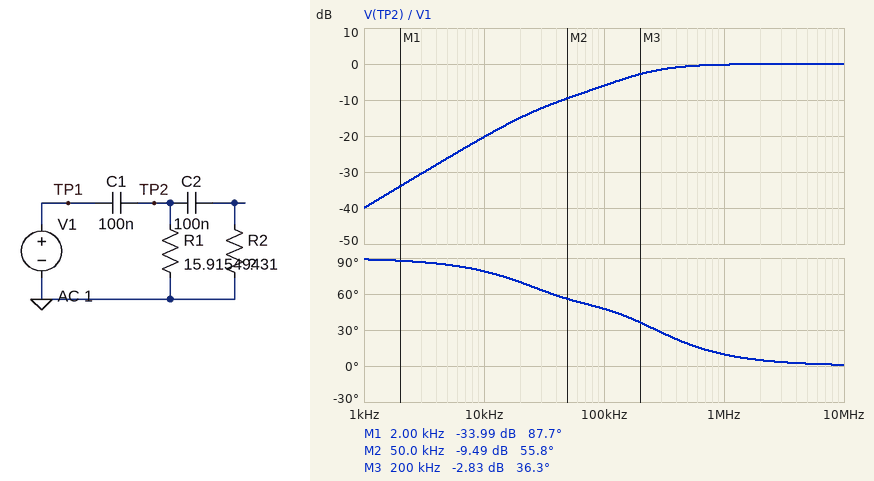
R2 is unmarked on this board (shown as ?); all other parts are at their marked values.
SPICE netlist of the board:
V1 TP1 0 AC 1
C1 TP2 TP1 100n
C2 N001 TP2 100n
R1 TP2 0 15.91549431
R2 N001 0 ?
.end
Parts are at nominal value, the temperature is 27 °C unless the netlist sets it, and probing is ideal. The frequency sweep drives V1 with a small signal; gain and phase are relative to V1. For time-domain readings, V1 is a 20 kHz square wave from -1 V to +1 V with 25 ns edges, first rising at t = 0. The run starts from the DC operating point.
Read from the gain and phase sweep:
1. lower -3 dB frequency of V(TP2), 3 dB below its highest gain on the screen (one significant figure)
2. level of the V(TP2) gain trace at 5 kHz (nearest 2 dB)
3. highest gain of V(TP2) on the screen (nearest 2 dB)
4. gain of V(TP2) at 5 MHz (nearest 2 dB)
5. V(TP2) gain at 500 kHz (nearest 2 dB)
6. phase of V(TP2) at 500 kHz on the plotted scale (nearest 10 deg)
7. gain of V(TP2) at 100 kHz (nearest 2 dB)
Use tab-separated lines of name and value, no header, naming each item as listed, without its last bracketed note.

lower -3 dB frequency of V(TP2), 3 dB below its highest gain on the screen	200 kHz
level of the V(TP2) gain trace at 5 kHz	-26 dB
highest gain of V(TP2) on the screen	0 dB
gain of V(TP2) at 5 MHz	0 dB
V(TP2) gain at 500 kHz	0 dB
phase of V(TP2) at 500 kHz on the plotted scale	20 deg
gain of V(TP2) at 100 kHz	-6 dB
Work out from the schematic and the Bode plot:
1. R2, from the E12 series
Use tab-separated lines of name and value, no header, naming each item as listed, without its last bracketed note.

R2, from the E12 series	22 Ω
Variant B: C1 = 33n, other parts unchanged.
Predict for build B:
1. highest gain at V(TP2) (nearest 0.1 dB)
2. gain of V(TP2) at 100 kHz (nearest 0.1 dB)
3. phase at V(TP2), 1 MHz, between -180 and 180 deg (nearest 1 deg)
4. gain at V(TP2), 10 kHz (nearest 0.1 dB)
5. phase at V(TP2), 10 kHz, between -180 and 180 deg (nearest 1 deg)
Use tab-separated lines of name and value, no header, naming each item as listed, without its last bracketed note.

highest gain at V(TP2)	0 dB
gain of V(TP2) at 100 kHz	-13.8 dB
phase at V(TP2), 1 MHz, between -180 and 180 deg	27 deg
gain at V(TP2), 10 kHz	-29.8 dB
phase at V(TP2), 10 kHz, between -180 and 180 deg	83 deg
